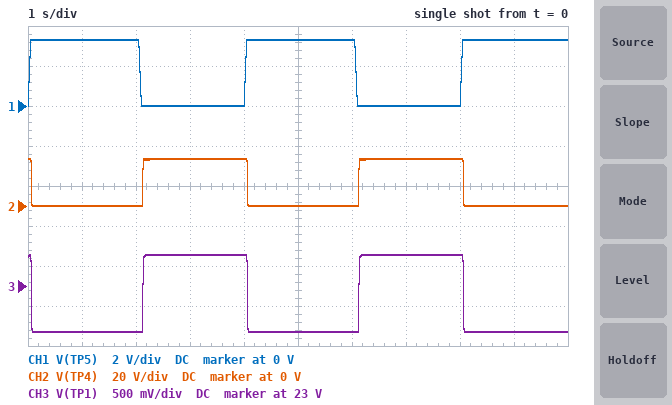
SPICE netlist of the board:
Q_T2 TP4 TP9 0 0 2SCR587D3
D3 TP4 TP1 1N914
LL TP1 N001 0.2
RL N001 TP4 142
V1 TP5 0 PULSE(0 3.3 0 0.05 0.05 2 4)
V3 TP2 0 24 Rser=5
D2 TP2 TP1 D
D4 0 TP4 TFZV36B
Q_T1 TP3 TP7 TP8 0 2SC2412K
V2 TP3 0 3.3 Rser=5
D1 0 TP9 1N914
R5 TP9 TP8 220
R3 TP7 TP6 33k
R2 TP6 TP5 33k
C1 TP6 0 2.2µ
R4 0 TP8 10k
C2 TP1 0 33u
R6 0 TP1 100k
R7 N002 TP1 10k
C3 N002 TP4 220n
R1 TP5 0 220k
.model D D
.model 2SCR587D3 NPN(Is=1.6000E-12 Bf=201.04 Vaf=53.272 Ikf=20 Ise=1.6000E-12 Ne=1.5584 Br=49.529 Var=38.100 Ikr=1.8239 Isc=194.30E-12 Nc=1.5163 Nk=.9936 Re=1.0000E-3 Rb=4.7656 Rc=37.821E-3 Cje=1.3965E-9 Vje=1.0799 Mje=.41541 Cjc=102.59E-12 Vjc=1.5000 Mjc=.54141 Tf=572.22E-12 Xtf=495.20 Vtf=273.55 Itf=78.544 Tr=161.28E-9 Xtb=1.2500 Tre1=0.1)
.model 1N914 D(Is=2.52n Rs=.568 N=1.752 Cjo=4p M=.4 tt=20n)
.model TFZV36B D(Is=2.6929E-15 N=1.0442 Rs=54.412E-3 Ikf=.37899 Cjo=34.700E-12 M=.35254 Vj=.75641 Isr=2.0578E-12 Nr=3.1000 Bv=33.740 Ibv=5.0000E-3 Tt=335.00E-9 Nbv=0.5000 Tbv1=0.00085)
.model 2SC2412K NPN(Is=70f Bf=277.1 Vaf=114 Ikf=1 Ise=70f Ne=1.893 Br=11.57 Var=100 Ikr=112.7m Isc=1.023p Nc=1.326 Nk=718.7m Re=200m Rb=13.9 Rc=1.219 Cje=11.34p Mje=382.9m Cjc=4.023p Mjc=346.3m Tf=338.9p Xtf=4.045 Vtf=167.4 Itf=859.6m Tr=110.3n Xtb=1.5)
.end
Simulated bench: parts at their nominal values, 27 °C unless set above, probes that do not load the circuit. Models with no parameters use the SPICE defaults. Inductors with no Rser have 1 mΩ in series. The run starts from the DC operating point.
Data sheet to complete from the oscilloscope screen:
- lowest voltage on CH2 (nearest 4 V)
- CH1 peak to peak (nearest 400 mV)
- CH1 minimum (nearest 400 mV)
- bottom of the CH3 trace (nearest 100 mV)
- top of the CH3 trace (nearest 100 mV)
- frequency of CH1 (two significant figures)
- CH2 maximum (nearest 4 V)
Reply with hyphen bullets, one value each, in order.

- 0 V
- 3.2 V
- 0 V
- 22.4 V
- 23.4 V
- 250 mHz
- 24 V
